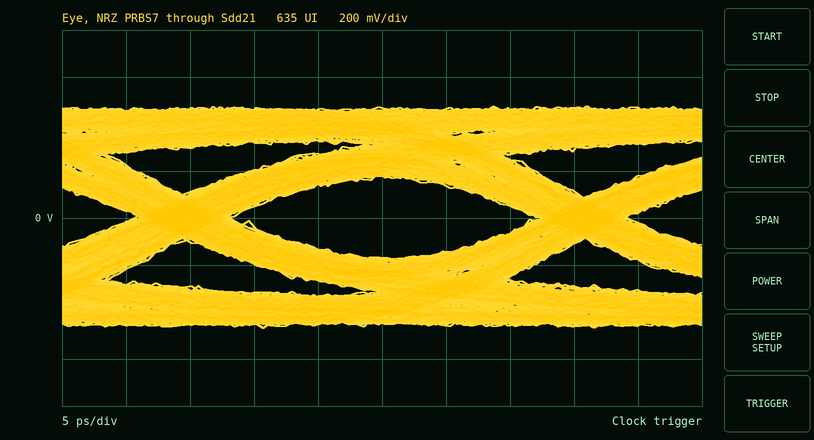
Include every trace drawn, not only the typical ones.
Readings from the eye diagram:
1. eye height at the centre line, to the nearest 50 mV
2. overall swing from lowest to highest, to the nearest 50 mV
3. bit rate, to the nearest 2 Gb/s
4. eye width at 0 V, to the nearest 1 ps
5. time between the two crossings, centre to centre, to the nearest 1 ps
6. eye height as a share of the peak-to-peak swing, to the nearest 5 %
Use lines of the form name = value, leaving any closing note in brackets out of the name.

eye height at the centre line, to the nearest 50 mV = 350 mV
overall swing from lowest to highest, to the nearest 50 mV = 950 mV
bit rate, to the nearest 2 Gb/s = 32 Gb/s
eye width at 0 V, to the nearest 1 ps = 24 ps
time between the two crossings, centre to centre, to the nearest 1 ps = 31 ps
eye height as a share of the peak-to-peak swing, to the nearest 5 % = 35 %
